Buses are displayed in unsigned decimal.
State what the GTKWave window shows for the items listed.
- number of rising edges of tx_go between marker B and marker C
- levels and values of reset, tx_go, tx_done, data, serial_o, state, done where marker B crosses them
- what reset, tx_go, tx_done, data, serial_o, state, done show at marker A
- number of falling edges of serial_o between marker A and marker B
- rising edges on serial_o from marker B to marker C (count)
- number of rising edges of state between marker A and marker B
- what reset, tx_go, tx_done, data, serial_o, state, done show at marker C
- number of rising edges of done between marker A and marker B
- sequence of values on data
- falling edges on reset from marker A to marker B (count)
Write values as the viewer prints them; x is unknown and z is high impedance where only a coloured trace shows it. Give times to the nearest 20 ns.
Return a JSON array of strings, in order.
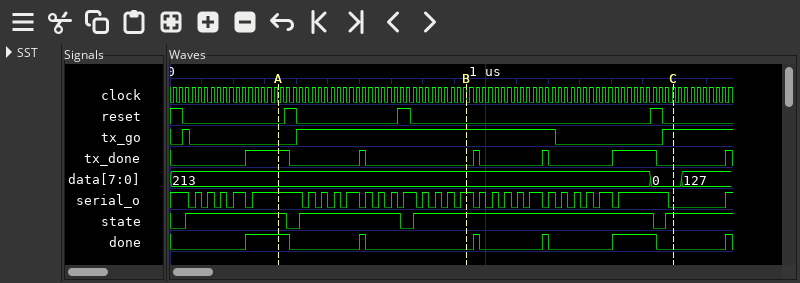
["1", "reset=0, tx_go=1, tx_done=0, data=213, serial_o=1, state=1, done=0", "reset=0, tx_go=0, tx_done=1, data=213, serial_o=1, state=1, done=1", "12", "11", "2", "reset=0, tx_go=1, tx_done=0, data=0, serial_o=0, state=1, done=0", "1", "213, 0, 127", "2"]
